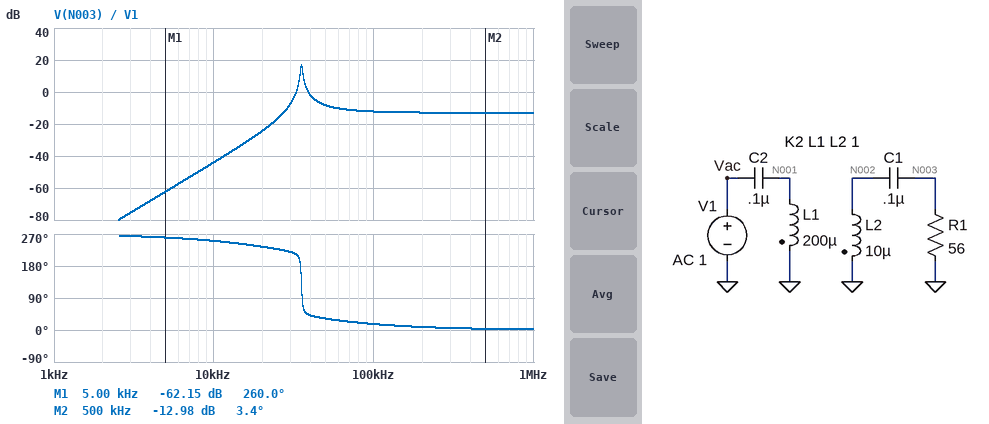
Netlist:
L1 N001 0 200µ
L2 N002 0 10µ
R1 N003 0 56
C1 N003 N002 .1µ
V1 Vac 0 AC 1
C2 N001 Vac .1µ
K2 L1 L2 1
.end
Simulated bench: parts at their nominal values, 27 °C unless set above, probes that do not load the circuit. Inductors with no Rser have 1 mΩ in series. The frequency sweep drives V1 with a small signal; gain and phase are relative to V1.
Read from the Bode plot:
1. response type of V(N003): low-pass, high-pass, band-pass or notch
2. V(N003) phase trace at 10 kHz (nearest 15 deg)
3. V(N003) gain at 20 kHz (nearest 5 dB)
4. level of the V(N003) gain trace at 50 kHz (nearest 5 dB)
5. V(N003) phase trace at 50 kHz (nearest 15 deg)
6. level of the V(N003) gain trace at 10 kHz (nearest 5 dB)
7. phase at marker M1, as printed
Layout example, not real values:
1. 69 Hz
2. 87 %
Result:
1. high-pass
2. 255 deg
3. -25 dB
4. -10 dB
5. 30 deg
6. -45 dB
7. 260.0 deg
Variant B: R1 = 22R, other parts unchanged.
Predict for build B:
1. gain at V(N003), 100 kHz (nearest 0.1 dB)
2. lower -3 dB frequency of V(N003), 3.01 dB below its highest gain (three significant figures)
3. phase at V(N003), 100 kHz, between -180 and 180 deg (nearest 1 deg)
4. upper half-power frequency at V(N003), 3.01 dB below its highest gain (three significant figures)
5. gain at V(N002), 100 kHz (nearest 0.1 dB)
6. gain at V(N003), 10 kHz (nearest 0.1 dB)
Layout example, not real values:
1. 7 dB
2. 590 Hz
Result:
1. -13.8 dB
2. 34.6 kHz
3. 37 deg
4. 35.2 kHz
5. -12.0 dB
6. -51.6 dB
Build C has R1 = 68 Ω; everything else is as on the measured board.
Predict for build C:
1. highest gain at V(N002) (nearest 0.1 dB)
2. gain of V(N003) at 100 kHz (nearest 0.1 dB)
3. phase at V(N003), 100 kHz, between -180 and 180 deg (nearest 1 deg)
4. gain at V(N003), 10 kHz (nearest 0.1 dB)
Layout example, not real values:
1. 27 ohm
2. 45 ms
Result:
1. 19.7 dB
2. -12.1 dB
3. 14 deg
4. -42.4 dB
